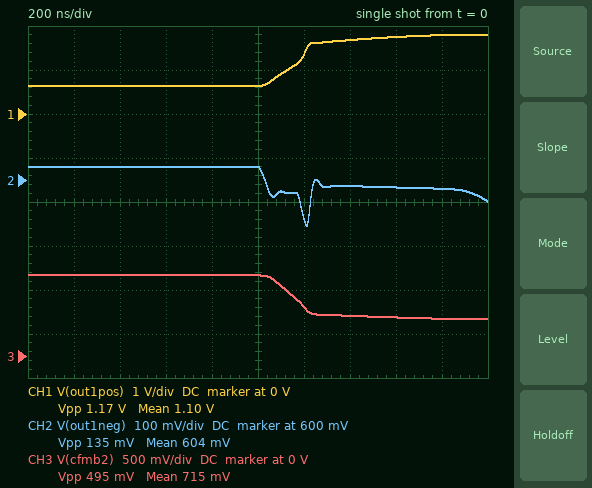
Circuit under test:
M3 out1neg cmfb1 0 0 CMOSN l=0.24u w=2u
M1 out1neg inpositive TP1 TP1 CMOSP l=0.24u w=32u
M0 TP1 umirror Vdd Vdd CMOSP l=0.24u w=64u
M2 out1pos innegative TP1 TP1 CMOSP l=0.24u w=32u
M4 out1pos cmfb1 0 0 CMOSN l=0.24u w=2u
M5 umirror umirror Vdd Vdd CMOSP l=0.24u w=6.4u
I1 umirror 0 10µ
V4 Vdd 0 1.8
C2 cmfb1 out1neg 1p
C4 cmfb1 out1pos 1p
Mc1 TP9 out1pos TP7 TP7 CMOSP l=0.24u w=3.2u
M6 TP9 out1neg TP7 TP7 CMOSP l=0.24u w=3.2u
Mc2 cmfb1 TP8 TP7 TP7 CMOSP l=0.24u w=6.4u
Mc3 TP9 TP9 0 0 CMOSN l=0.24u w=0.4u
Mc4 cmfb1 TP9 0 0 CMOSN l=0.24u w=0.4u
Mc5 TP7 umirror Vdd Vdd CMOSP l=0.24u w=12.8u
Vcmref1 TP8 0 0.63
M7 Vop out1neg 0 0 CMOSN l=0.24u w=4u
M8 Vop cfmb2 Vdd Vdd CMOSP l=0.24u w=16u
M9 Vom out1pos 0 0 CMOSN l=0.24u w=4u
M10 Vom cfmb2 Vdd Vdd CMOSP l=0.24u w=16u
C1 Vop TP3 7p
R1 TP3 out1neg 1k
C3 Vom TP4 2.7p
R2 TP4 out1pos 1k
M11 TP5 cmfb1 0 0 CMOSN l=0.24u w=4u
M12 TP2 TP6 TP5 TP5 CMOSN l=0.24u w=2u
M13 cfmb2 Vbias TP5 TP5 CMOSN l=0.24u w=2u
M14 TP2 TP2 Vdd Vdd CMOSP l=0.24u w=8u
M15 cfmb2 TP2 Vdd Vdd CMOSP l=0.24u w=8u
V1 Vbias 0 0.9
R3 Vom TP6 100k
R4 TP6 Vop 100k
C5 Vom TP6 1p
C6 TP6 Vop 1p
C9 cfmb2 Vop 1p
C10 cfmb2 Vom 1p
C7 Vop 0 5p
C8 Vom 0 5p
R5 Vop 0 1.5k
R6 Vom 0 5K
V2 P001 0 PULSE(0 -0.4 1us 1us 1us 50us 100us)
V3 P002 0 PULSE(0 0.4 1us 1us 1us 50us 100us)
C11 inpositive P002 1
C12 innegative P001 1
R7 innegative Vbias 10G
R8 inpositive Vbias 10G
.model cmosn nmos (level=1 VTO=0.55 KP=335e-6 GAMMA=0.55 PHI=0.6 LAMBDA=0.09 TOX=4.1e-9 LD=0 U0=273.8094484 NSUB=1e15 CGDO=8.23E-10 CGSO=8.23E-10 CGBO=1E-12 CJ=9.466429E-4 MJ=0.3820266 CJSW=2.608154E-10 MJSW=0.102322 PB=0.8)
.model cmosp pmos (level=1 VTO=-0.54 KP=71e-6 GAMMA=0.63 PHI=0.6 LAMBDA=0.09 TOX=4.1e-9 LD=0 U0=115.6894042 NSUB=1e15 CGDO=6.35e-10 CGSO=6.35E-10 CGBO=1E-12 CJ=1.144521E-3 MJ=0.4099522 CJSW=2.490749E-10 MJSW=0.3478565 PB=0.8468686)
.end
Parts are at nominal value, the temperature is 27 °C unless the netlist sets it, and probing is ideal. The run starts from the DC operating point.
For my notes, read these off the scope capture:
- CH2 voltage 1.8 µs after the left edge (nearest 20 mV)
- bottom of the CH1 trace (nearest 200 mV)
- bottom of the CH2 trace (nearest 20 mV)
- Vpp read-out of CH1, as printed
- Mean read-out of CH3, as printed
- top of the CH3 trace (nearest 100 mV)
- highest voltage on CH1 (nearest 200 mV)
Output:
580 mV
600 mV
500 mV
1.17 V
715 mV
900 mV
1.8 V
